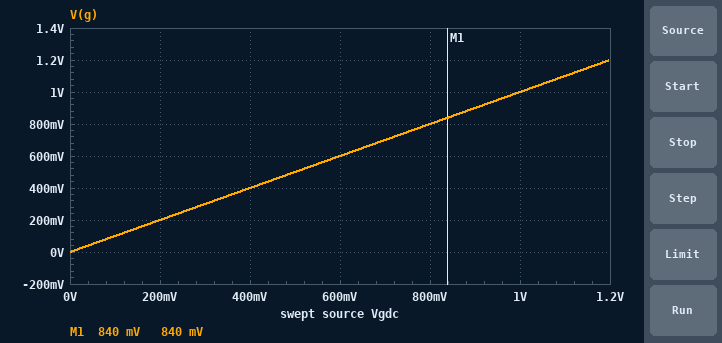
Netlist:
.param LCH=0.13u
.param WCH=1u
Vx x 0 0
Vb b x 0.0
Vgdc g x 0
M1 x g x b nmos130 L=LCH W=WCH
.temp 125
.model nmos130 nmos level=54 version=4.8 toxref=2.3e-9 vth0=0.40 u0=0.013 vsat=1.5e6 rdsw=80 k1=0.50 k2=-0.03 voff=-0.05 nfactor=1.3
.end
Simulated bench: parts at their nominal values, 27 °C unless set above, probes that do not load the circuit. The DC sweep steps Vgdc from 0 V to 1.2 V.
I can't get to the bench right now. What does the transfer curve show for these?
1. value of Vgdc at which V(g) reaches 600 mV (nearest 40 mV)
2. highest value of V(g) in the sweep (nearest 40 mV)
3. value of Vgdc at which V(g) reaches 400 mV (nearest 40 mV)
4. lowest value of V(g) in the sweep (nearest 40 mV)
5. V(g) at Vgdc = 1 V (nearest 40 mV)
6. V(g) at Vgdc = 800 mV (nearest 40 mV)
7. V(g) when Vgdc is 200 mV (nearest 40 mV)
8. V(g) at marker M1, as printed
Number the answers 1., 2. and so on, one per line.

1. 600 mV
2. 1.20 V
3. 400 mV
4. 0 V
5. 1.00 V
6. 800 mV
7. 200 mV
8. 840 mV
